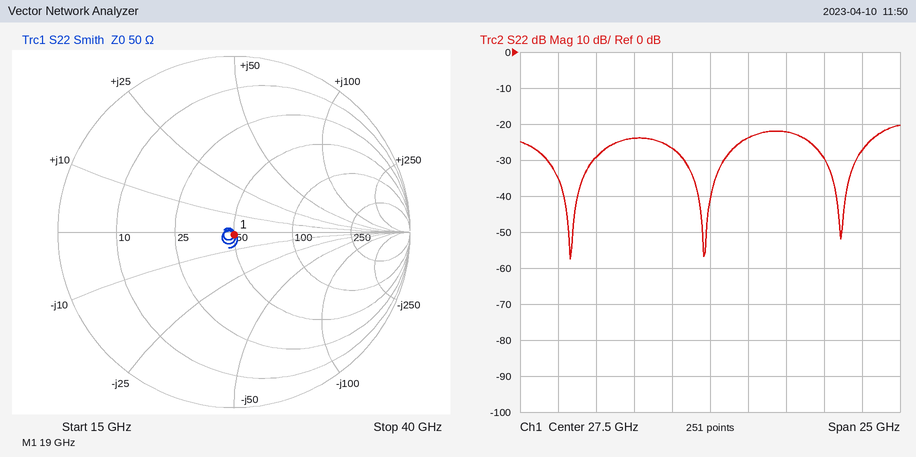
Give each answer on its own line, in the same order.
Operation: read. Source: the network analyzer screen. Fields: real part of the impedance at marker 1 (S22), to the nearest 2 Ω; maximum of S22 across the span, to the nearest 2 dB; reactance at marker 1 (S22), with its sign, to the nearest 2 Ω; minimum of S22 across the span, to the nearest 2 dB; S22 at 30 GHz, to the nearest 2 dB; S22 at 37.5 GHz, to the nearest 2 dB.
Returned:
50 Ω
-20 dB
-2 Ω
-58 dB
-24 dB
-28 dB
